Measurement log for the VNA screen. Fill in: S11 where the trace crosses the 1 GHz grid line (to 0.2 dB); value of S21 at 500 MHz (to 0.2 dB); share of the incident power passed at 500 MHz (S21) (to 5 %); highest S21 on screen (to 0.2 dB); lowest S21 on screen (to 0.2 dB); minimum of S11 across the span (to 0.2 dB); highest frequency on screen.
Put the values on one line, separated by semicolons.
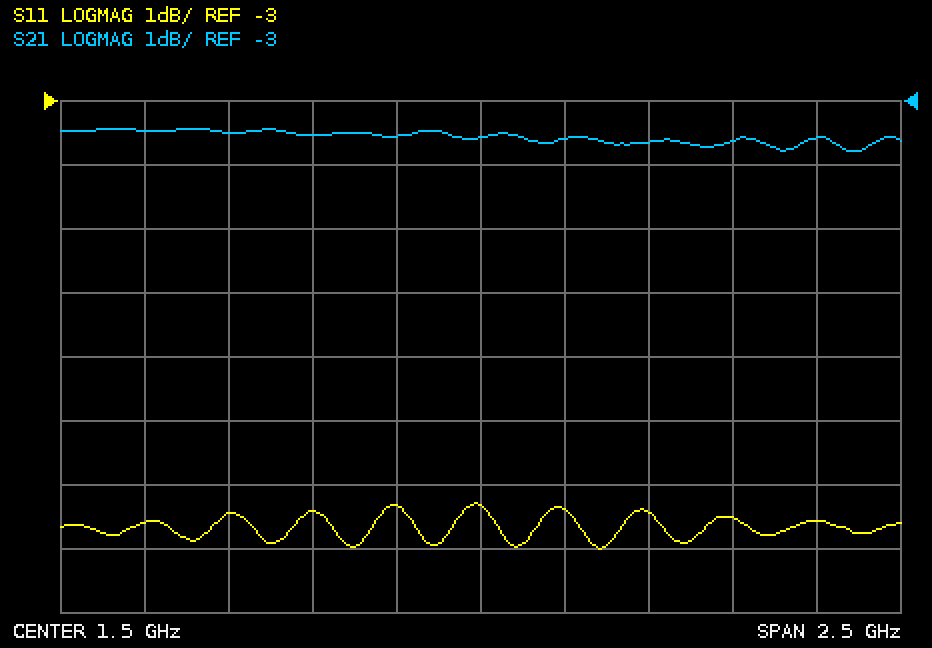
-9.4 dB; -3.4 dB; 45 %; -3.4 dB; -3.8 dB; -10.0 dB; 2.75 GHz
